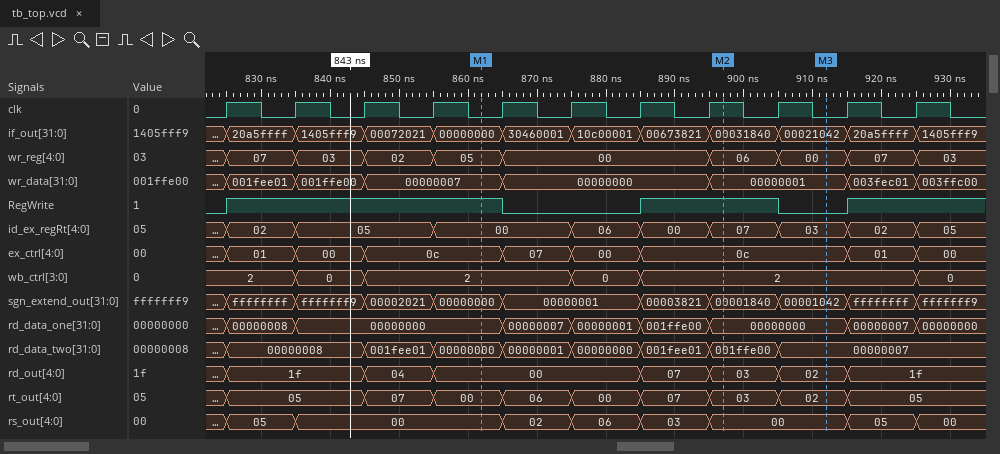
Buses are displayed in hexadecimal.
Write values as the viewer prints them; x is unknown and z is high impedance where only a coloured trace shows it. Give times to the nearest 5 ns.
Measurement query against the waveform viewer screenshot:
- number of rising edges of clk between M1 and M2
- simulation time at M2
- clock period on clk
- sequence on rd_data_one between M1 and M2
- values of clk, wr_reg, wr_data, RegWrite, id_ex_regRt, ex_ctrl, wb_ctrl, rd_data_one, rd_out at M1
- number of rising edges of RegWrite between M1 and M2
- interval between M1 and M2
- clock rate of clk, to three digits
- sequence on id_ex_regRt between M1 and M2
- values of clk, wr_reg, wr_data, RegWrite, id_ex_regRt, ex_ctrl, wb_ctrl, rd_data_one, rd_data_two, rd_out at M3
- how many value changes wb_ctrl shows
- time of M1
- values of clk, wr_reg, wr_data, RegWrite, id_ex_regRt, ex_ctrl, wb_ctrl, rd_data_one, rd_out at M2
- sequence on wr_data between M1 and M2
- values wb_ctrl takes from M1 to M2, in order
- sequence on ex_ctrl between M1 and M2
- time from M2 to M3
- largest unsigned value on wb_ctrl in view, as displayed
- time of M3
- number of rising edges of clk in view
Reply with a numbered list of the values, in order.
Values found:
1. 4
2. 895 ns
3. 10 ns
4. 00000000, 00000007, 00000001, 001ffe00, 00000000
5. clk=0, wr_reg=05, wr_data=00000007, RegWrite=1, id_ex_regRt=00, ex_ctrl=0c, wb_ctrl=2, rd_data_one=00000000, rd_out=00
6. 1
7. 35 ns
8. 100 MHz
9. 00, 06, 00, 07
10. clk=0, wr_reg=00, wr_data=00000001, RegWrite=0, id_ex_regRt=03, ex_ctrl=0c, wb_ctrl=2, rd_data_one=00000000, rd_data_two=00000007, rd_out=02
11. 5
12. 860 ns
13. clk=1, wr_reg=06, wr_data=00000001, RegWrite=1, id_ex_regRt=07, ex_ctrl=0c, wb_ctrl=2, rd_data_one=00000000, rd_out=03
14. 00000007, 00000000, 00000001
15. 2, 0, 2
16. 0c, 07, 00, 0c
17. 15 ns
18. 2
19. 910 ns
20. 11
